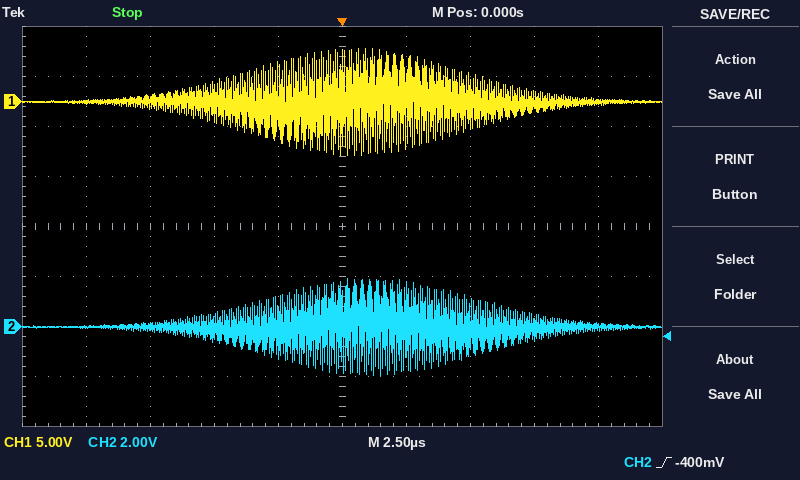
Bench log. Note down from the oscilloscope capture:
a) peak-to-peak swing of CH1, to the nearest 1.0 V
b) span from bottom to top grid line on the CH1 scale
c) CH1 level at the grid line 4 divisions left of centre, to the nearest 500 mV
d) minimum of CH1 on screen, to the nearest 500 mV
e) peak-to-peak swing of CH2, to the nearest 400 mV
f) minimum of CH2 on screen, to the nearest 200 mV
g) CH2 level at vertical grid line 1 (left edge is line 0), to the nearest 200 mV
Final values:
11.0 V
40 V
0.0 V
-5.5 V
4.0 V
-2.0 V
0.0 V
